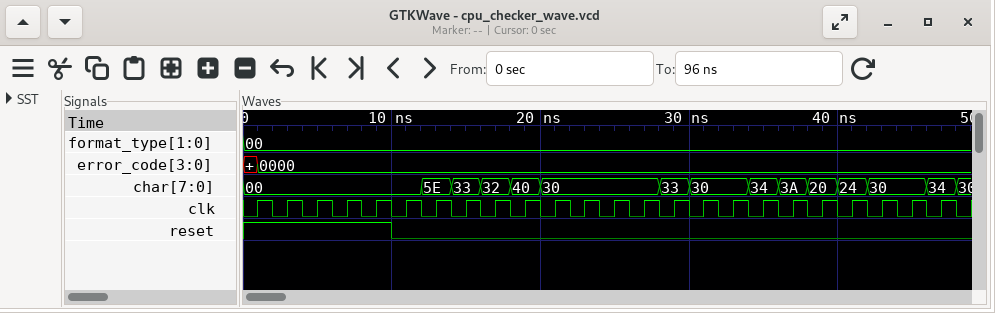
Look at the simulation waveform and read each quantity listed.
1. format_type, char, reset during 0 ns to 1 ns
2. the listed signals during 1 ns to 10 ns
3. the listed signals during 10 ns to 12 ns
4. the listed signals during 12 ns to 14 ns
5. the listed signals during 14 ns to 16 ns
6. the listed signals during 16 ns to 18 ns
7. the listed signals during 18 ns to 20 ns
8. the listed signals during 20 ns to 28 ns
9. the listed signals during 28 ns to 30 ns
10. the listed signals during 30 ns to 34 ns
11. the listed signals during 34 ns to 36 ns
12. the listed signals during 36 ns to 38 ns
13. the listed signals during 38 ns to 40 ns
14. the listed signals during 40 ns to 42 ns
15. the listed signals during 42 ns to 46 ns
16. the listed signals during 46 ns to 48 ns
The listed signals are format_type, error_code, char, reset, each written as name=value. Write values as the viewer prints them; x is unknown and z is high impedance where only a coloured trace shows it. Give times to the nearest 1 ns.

format_type=00, char=00, reset=1
format_type=00, error_code=0000, char=00, reset=1
format_type=00, error_code=0000, char=00, reset=0
format_type=00, error_code=0000, char=5E, reset=0
format_type=00, error_code=0000, char=33, reset=0
format_type=00, error_code=0000, char=32, reset=0
format_type=00, error_code=0000, char=40, reset=0
format_type=00, error_code=0000, char=30, reset=0
format_type=00, error_code=0000, char=33, reset=0
format_type=00, error_code=0000, char=30, reset=0
format_type=00, error_code=0000, char=34, reset=0
format_type=00, error_code=0000, char=3A, reset=0
format_type=00, error_code=0000, char=20, reset=0
format_type=00, error_code=0000, char=24, reset=0
format_type=00, error_code=0000, char=30, reset=0
format_type=00, error_code=0000, char=34, reset=0
